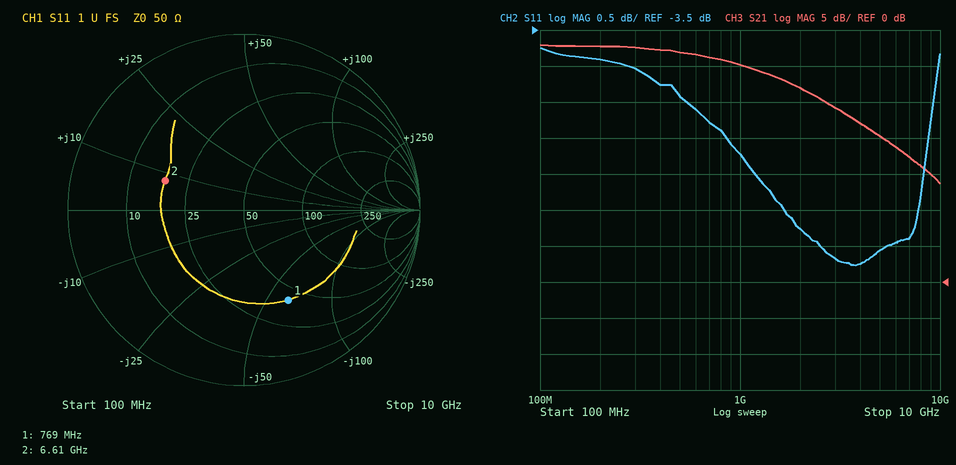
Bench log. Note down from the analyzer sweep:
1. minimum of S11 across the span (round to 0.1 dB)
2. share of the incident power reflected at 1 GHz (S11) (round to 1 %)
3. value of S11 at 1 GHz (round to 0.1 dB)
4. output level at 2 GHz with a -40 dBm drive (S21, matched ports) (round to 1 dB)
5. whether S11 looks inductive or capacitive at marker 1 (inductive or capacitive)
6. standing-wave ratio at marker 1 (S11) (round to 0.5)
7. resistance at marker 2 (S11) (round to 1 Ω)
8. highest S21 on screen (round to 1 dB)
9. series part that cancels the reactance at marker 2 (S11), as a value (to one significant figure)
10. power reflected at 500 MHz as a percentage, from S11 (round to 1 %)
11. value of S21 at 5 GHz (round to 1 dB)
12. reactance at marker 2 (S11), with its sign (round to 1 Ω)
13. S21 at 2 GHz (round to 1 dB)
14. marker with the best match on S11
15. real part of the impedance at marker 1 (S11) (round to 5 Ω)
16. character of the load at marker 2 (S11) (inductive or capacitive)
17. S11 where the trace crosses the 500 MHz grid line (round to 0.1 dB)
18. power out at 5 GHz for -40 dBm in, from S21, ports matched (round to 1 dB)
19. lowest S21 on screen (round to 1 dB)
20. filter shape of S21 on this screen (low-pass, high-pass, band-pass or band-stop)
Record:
-6.8 dB
30 %
-5.2 dB
-13 dBm
capacitive
3.5
18 Ω
33 dB
3 pF
36 %
20 dB
+8 Ω
27 dB
marker 2
40 Ω
inductive
-4.4 dB
-20 dBm
14 dB
low-pass
